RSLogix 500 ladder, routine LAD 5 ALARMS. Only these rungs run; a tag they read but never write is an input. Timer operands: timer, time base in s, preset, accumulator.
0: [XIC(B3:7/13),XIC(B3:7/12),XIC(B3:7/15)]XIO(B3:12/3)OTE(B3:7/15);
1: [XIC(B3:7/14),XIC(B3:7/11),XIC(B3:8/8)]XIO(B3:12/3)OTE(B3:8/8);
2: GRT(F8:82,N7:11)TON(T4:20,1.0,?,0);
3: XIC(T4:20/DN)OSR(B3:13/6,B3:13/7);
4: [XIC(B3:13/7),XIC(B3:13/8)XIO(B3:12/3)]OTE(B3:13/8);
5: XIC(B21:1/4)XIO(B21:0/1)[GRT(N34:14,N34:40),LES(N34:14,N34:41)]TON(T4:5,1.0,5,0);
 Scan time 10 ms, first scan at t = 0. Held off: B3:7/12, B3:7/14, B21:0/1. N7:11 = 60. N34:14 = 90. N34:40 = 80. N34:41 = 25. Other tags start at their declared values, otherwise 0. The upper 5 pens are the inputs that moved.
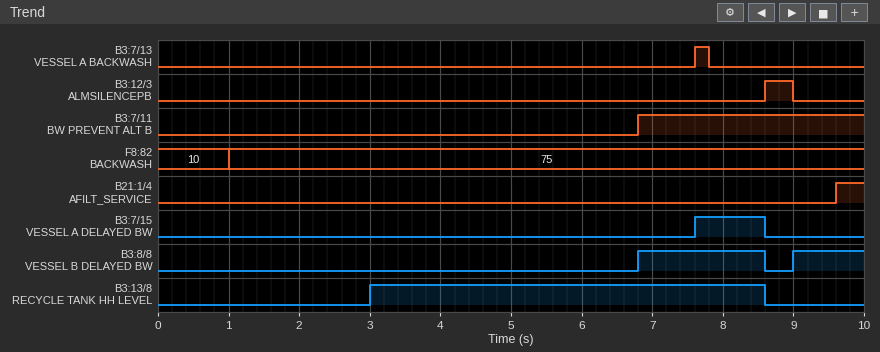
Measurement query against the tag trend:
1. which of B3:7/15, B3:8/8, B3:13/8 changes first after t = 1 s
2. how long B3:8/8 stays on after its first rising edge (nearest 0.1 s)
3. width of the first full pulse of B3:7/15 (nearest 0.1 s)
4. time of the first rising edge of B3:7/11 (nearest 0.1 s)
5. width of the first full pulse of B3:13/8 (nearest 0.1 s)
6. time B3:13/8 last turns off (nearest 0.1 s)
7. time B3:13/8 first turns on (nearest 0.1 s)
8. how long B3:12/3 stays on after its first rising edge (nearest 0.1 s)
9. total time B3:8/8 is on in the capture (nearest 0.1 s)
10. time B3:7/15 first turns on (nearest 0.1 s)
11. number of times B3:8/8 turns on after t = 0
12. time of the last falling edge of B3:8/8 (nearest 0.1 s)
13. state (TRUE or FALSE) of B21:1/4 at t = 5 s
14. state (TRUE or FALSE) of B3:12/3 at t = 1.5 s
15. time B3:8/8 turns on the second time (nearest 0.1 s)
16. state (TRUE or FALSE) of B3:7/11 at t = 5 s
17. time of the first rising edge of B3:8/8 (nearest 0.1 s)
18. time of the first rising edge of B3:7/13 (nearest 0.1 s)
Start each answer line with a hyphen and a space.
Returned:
- B3:13/8
- 1.8 s
- 1.0 s
- 6.8 s
- 5.6 s
- 8.6 s
- 3.0 s
- 0.4 s
- 2.8 s
- 7.6 s
- 2
- 8.6 s
- FALSE
- FALSE
- 9.0 s
- FALSE
- 6.8 s
- 7.6 s
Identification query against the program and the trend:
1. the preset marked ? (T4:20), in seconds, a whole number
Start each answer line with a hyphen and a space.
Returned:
- 2 s
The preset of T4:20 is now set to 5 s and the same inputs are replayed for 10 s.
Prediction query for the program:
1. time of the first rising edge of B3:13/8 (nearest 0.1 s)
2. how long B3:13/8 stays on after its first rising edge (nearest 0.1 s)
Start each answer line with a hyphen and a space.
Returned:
- 6.0 s
- 2.6 s
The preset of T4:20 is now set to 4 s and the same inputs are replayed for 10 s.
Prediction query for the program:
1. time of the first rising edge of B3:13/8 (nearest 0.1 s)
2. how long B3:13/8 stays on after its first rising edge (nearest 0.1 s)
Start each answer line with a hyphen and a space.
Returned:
- 5.0 s
- 3.6 s
